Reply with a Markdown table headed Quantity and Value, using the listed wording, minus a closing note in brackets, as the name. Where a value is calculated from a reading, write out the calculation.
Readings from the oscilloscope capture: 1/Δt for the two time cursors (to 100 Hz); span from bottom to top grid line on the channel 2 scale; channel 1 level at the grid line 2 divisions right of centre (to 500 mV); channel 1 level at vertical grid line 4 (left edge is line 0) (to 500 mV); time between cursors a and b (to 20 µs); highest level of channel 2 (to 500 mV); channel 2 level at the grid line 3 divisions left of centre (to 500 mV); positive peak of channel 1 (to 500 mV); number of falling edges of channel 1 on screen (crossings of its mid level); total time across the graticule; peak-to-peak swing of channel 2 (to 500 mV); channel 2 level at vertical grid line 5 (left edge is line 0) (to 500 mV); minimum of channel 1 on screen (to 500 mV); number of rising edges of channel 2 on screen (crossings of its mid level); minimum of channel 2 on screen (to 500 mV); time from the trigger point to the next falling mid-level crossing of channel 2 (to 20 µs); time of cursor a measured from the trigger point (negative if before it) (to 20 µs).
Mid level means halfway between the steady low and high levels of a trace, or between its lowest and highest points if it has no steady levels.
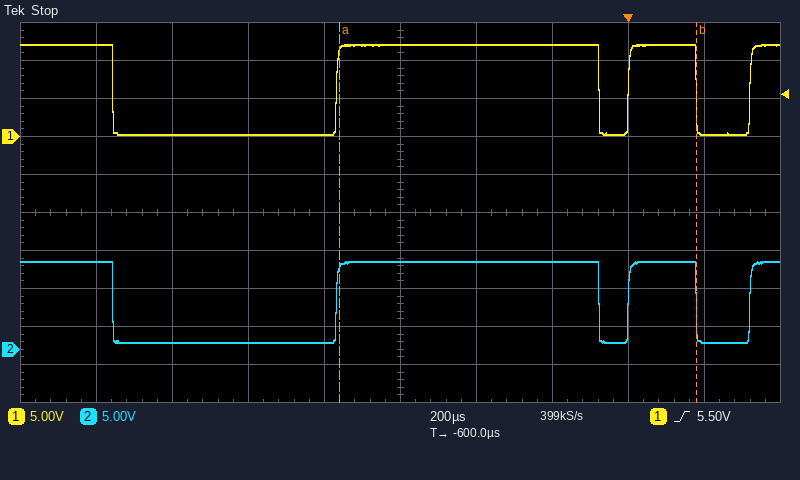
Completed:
| Quantity | Value |
|---|---|
| 1/Δt for the two time cursors | 1 / 940 µs ≈ 1.1 kHz |
| span from bottom to top grid line on the channel 2 scale | 50 V |
| channel 1 level at the grid line 2 divisions right of centre | 12.0 V |
| channel 1 level at vertical grid line 4 (left edge is line 0) | 500 mV |
| time between cursors a and b | 940 µs |
| highest level of channel 2 | 11.5 V |
| channel 2 level at the grid line 3 divisions left of centre | 1.0 V |
| positive peak of channel 1 | 12.0 V |
| number of falling edges of channel 1 on screen | 3 |
| total time across the graticule | 2 ms |
| peak-to-peak swing of channel 2 | 11.5 V − (1.0 V) = 10.5 V |
| channel 2 level at vertical grid line 5 (left edge is line 0) | 11.5 V |
| minimum of channel 1 on screen | 500 mV |
| number of rising edges of channel 2 on screen | 3 |
| minimum of channel 2 on screen | 1.0 V |
| time from the trigger point to the next falling mid-level crossing of channel 2 | 180 µs |
| time of cursor a measured from the trigger point (negative if before it) | -760 µs |
